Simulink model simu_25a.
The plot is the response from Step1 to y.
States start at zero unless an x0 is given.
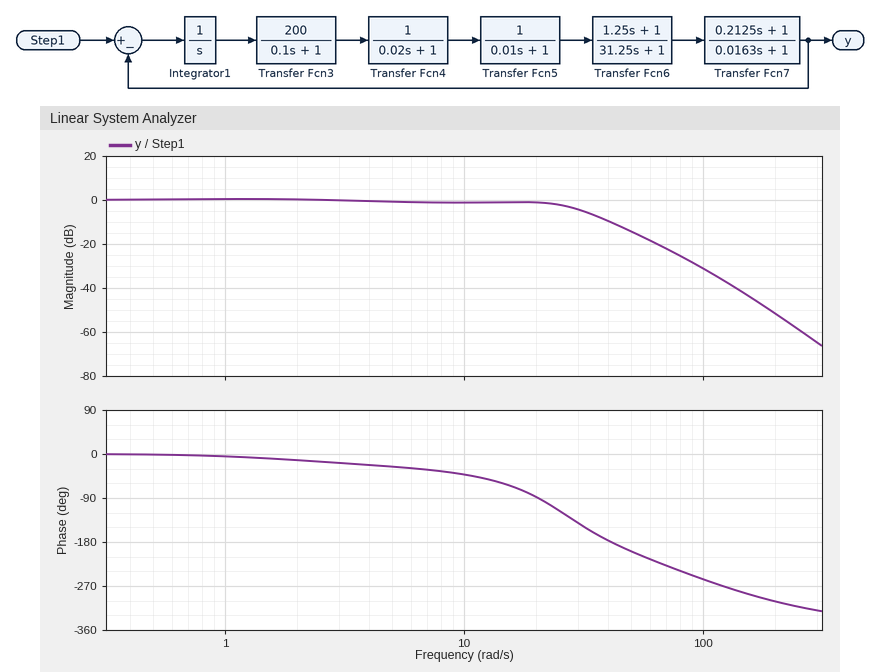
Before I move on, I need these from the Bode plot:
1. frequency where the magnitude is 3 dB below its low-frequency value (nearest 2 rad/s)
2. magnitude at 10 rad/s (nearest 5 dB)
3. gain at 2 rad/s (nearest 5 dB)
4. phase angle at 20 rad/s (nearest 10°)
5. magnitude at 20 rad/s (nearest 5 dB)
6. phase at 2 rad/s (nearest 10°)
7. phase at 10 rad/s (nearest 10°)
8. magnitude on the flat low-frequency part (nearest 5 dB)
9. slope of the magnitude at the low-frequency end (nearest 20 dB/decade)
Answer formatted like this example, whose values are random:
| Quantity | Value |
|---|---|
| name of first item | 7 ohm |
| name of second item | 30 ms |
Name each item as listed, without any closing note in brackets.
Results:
| Quantity | Value |
|---|---|
| frequency where the magnitude is 3 dB below its low-frequency value | 26 rad/s |
| magnitude at 10 rad/s | 0 dB |
| gain at 2 rad/s | 0 dB |
| phase angle at 20 rad/s | -90° |
| magnitude at 20 rad/s | 0 dB |
| phase at 2 rad/s | -10° |
| phase at 10 rad/s | -40° |
| magnitude on the flat low-frequency part | 0 dB |
| slope of the magnitude at the low-frequency end | 0 dB/decade |
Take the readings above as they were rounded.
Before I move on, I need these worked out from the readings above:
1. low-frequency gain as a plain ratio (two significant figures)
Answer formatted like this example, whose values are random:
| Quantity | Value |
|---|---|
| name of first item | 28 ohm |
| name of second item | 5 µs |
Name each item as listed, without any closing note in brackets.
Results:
| Quantity | Value |
|---|---|
| low-frequency gain as a plain ratio | 1.0 |
